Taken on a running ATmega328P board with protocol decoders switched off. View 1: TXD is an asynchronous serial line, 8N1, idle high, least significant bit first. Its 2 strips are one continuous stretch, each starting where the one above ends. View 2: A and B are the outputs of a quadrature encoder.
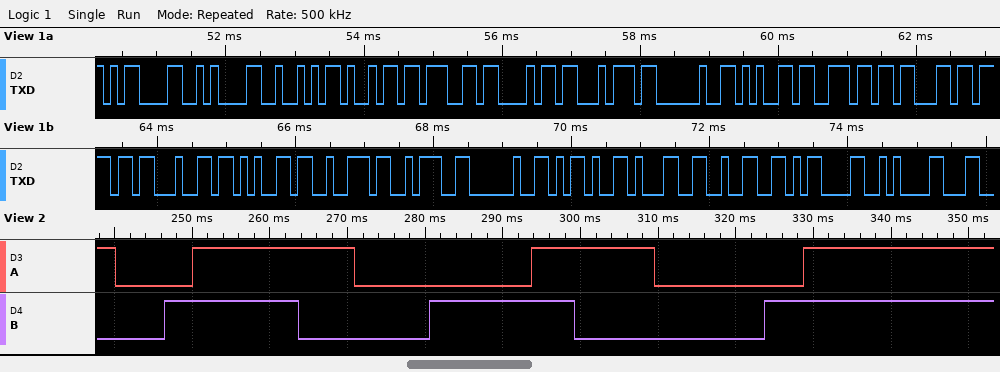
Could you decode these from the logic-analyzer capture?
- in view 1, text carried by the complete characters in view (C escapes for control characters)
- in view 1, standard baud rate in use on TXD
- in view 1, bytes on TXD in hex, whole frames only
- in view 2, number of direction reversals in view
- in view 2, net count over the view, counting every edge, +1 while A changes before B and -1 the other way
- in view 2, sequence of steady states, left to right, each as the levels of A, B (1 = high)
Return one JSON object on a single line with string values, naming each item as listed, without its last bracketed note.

{"in view 1, text carried by the complete characters in view": "\"\\r\\nRight encoder: -12\\r\\n\"", "in view 1, standard baud rate in use on TXD": "9600 baud", "in view 1, bytes on TXD in hex, whole frames only": "0x0D 0x0A 0x52 0x69 0x67 0x68 0x74 0x20 0x65 0x6E 0x63 0x6F 0x64 0x65 0x72 0x3A 0x20 0x2D 0x31 0x32 0x0D 0x0A", "in view 2, number of direction reversals in view": "0", "in view 2, net count over the view, counting every edge, +1 while A changes before B and -1 the other way": "-11", "in view 2, sequence of steady states, left to right, each as the levels of A, B": "10 00 01 11 10 00 01 11 10 00 01 11"}
